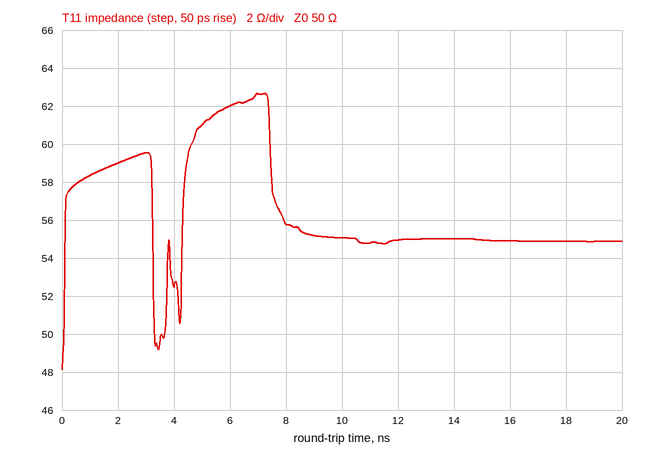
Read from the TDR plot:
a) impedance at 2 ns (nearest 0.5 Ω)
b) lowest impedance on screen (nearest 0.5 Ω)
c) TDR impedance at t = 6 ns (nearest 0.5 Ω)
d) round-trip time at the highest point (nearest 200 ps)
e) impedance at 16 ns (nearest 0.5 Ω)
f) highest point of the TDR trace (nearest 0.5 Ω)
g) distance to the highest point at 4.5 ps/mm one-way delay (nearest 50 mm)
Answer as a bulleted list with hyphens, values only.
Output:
- 59.0 Ω
- 48.0 Ω
- 62.0 Ω
- 7.2 ns
- 55.0 Ω
- 62.5 Ω
- 800 mm
